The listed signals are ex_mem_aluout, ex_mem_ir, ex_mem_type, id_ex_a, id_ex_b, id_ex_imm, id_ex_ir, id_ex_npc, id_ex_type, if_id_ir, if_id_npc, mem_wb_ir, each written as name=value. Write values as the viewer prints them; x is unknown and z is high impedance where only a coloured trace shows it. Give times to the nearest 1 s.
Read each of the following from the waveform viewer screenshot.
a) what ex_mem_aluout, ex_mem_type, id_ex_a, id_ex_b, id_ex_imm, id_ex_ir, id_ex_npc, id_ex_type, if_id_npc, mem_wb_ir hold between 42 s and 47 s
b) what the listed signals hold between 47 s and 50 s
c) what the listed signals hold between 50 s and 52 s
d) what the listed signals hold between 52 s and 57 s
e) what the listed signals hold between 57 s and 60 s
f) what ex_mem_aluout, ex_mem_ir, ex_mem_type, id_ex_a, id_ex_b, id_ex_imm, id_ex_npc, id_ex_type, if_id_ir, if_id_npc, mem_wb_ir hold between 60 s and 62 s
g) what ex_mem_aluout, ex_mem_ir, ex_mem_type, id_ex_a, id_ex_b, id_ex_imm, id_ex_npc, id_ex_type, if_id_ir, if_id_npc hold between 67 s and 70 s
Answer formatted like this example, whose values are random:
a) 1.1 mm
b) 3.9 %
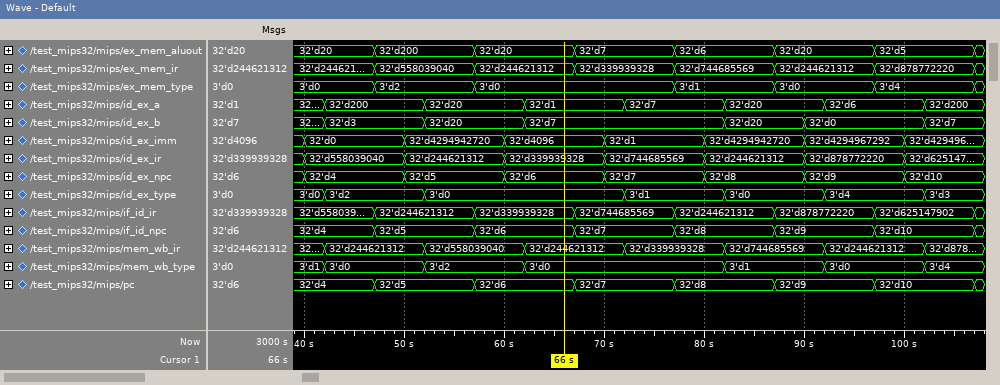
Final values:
a) ex_mem_aluout=32'd20, ex_mem_type=3'd0, id_ex_a=32'd200, id_ex_b=32'd3, id_ex_imm=32'd0, id_ex_ir=32'd558039040, id_ex_npc=32'd4, id_ex_type=3'd2, if_id_npc=32'd4, mem_wb_ir=32'd244621312
b) ex_mem_aluout=32'd200, ex_mem_ir=32'd558039040, ex_mem_type=3'd2, id_ex_a=32'd200, id_ex_b=32'd3, id_ex_imm=32'd0, id_ex_ir=32'd558039040, id_ex_npc=32'd4, id_ex_type=3'd2, if_id_ir=32'd244621312, if_id_npc=32'd5, mem_wb_ir=32'd244621312
c) ex_mem_aluout=32'd200, ex_mem_ir=32'd558039040, ex_mem_type=3'd2, id_ex_a=32'd200, id_ex_b=32'd3, id_ex_imm=32'd4294942720, id_ex_ir=32'd244621312, id_ex_npc=32'd5, id_ex_type=3'd2, if_id_ir=32'd244621312, if_id_npc=32'd5, mem_wb_ir=32'd244621312
d) ex_mem_aluout=32'd200, ex_mem_ir=32'd558039040, ex_mem_type=3'd2, id_ex_a=32'd20, id_ex_b=32'd20, id_ex_imm=32'd4294942720, id_ex_ir=32'd244621312, id_ex_npc=32'd5, id_ex_type=3'd0, if_id_ir=32'd244621312, if_id_npc=32'd5, mem_wb_ir=32'd558039040
e) ex_mem_aluout=32'd20, ex_mem_ir=32'd244621312, ex_mem_type=3'd0, id_ex_a=32'd20, id_ex_b=32'd20, id_ex_imm=32'd4294942720, id_ex_ir=32'd244621312, id_ex_npc=32'd5, id_ex_type=3'd0, if_id_ir=32'd339939328, if_id_npc=32'd6, mem_wb_ir=32'd558039040
f) ex_mem_aluout=32'd20, ex_mem_ir=32'd244621312, ex_mem_type=3'd0, id_ex_a=32'd20, id_ex_b=32'd20, id_ex_imm=32'd4096, id_ex_npc=32'd6, id_ex_type=3'd0, if_id_ir=32'd339939328, if_id_npc=32'd6, mem_wb_ir=32'd558039040
g) ex_mem_aluout=32'd7, ex_mem_ir=32'd339939328, ex_mem_type=3'd0, id_ex_a=32'd1, id_ex_b=32'd7, id_ex_imm=32'd4096, id_ex_npc=32'd6, id_ex_type=3'd0, if_id_ir=32'd744685569, if_id_npc=32'd7
